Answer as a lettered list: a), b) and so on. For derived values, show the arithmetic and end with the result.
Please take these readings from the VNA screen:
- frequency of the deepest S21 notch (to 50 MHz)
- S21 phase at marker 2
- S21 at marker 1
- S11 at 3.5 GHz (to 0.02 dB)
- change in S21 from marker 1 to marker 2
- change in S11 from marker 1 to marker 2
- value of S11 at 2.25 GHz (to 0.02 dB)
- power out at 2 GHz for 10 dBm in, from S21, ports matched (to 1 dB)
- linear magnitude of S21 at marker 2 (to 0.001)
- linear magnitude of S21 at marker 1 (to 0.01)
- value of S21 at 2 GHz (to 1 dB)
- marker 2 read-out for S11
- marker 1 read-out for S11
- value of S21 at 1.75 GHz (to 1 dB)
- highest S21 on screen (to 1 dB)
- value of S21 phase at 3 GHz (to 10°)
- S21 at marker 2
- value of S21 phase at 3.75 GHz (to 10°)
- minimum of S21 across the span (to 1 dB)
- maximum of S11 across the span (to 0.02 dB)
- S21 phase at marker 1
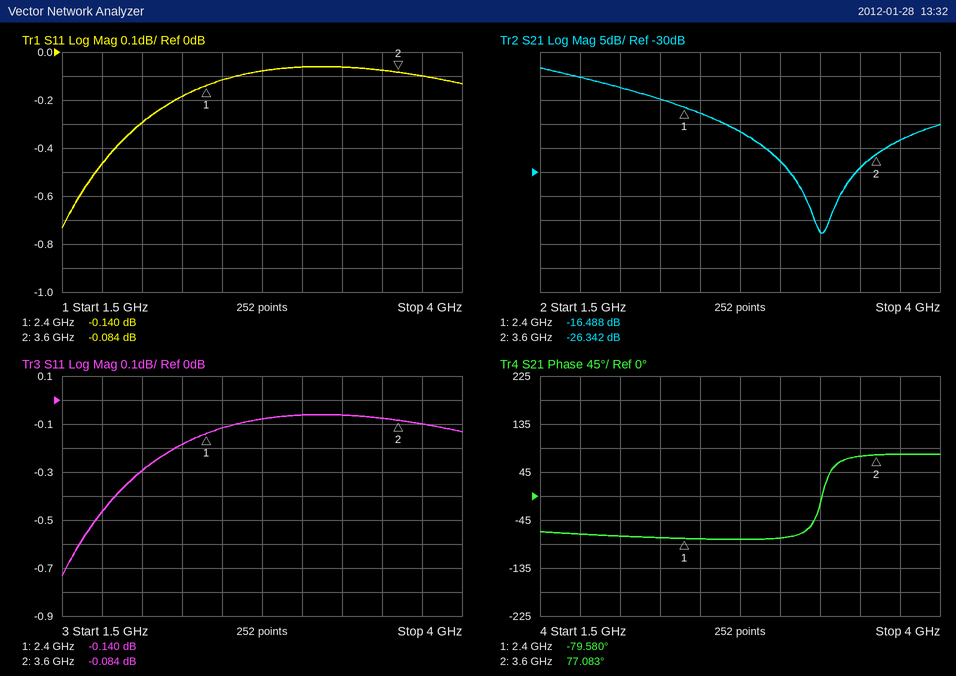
a) 3.25 GHz
b) 77.083°
c) -16.488 dB
d) -0.08 dB
e) -26.342 − (-16.488) = -9.854 dB
f) -0.084 − (-0.14) = 0.056 dB
g) -0.18 dB
h) 10 dBm + (-12 dB) = -2 dBm
i) 10^(-26.342/20) ≈ 0.048
j) 10^(-16.488/20) ≈ 0.15
k) -12 dB
l) -0.084 dB
m) -0.140 dB
n) -10 dB
o) -8 dB
p) -80°
q) -26.342 dB
r) 80°
s) -43 dB
t) -0.06 dB
u) -79.580°
